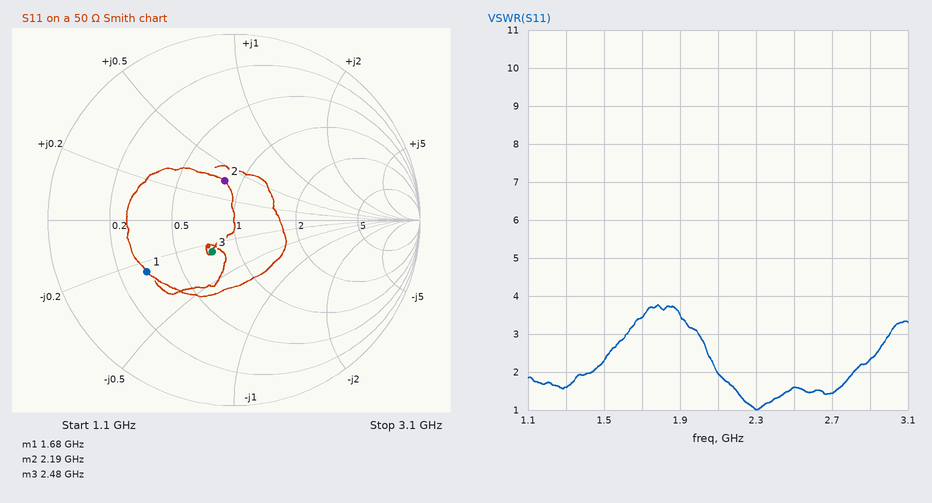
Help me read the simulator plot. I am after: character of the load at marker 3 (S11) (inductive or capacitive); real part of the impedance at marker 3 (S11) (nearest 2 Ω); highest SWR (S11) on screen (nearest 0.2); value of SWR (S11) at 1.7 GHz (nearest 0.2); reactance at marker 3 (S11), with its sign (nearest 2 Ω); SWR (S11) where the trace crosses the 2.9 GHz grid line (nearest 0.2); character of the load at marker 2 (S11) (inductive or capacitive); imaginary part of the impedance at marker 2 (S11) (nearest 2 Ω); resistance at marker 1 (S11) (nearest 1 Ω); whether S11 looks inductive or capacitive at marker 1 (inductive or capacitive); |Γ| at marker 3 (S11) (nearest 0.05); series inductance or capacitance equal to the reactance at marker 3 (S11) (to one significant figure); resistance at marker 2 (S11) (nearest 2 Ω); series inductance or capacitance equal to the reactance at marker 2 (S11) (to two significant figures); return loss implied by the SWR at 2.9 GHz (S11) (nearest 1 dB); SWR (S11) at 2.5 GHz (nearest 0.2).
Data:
capacitive
38 Ω
3.8
3.4
-14 Ω
2.4
inductive
+18 Ω
16 Ω
capacitive
0.20
5 pF
42 Ω
1.3 nH
8 dB
1.6
